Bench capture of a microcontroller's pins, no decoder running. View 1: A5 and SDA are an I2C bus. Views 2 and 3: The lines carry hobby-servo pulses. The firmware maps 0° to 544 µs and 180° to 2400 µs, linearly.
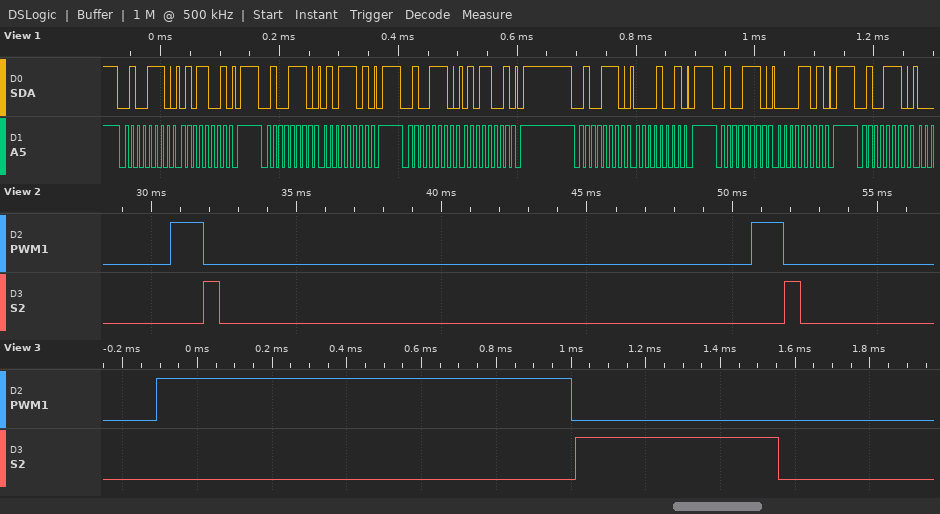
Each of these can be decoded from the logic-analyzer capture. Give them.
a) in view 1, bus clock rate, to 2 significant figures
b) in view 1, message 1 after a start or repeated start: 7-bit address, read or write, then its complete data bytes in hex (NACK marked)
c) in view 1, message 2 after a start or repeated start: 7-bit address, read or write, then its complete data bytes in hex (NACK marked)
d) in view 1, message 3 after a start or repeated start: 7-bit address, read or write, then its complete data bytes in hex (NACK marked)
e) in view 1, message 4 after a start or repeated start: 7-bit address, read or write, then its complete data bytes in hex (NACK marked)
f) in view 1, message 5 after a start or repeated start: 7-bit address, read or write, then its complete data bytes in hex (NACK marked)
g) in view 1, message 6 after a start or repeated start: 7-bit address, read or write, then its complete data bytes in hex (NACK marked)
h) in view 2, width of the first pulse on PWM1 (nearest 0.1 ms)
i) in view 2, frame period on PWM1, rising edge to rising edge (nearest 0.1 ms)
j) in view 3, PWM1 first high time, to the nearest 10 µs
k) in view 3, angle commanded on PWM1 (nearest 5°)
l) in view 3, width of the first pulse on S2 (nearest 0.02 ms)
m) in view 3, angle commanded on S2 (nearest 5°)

100 kHz
0x27 write: 59
0x27 write: 5D
0x27 write: 59
0x27 write: 09
0x27 write: 0D
0x27 write
1.1 ms
20.0 ms
1110 µs
55°
0.54 ms
0°
